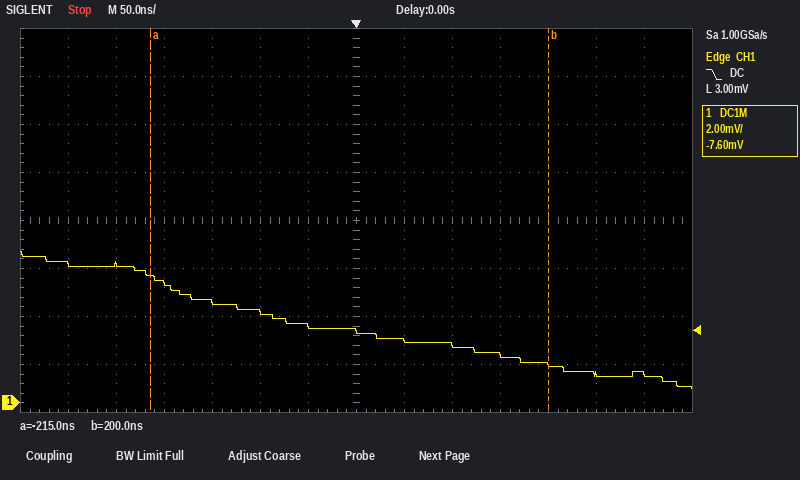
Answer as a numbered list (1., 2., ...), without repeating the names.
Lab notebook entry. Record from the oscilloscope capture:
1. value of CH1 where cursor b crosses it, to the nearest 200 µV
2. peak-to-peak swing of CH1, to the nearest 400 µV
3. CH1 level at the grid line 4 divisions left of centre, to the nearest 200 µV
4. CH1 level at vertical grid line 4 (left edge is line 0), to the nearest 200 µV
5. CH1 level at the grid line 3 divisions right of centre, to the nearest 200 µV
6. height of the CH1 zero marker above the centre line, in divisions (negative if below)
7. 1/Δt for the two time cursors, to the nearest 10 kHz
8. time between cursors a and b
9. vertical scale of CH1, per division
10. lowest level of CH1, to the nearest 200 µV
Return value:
1. 1.6 mV
2. 5.6 mV
3. 5.0 mV
4. 4.2 mV
5. 2.0 mV
6. -3.8 div
7. 2.41 MHz
8. 415 ns
9. 2 mV
10. 600 µV
